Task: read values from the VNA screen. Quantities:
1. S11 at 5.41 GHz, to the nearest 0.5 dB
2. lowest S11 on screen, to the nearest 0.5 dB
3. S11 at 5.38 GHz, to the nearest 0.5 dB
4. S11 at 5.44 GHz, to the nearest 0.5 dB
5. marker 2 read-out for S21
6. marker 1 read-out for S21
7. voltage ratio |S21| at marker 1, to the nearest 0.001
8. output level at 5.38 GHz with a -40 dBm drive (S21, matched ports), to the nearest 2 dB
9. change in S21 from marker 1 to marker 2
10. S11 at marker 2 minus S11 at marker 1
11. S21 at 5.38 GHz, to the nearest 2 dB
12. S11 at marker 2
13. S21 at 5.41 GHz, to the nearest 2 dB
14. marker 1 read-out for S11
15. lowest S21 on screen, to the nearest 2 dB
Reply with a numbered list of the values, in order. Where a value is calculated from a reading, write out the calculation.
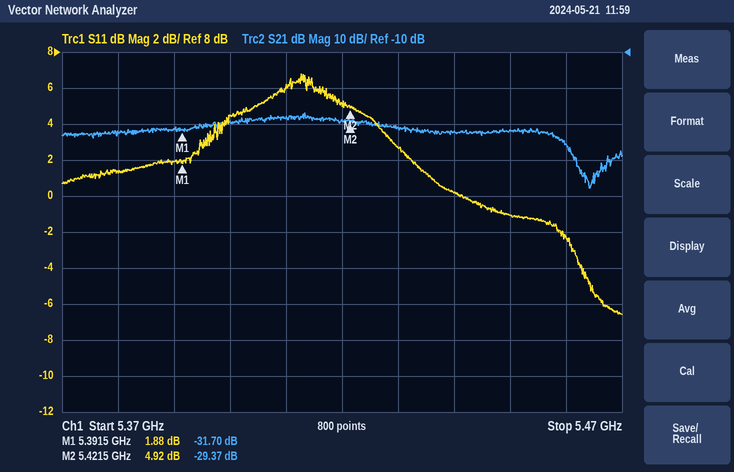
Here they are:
1. 6.0 dB
2. -6.5 dB
3. 1.5 dB
4. 0.0 dB
5. -29.37 dB
6. -31.70 dB
7. 10^(-31.7/20) ≈ 0.026
8. -40 dBm + (-32 dB) = -72 dBm
9. -29.37 − (-31.7) = 2.33 dB
10. 4.92 − (1.88) = 3.04 dB
11. -32 dB
12. 4.92 dB
13. -28 dB
14. 1.88 dB
15. -48 dB
